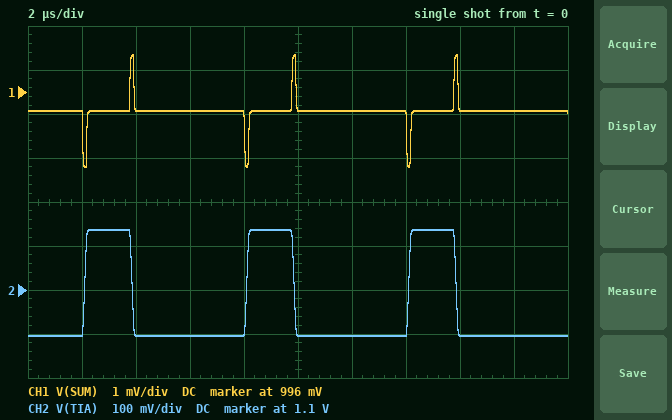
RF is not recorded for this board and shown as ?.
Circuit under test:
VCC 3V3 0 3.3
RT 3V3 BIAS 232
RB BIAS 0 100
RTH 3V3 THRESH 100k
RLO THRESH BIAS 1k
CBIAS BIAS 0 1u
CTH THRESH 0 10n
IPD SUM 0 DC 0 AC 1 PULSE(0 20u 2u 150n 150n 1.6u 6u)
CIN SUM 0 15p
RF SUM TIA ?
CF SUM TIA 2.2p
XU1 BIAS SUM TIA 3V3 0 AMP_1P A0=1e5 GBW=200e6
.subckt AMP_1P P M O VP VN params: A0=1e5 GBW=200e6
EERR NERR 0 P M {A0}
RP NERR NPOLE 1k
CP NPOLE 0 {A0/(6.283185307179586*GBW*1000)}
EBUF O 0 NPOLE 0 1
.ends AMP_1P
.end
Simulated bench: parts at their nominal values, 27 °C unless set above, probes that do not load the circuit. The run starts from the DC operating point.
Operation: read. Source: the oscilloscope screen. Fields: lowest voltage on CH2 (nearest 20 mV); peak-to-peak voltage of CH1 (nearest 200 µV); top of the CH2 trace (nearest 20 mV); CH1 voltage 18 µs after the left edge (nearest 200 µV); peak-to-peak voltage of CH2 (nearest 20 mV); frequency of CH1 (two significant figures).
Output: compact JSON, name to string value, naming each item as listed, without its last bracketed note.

{"lowest voltage on CH2": "1.00 V", "peak-to-peak voltage of CH1": "2.6 mV", "top of the CH2 trace": "1.24 V", "CH1 voltage 18 µs after the left edge": "995.6 mV", "peak-to-peak voltage of CH2": "240 mV", "frequency of CH1": "170 kHz"}
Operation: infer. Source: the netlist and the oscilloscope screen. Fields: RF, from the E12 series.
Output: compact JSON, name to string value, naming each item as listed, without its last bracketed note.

{"RF, from the E12 series": "12 kΩ"}
